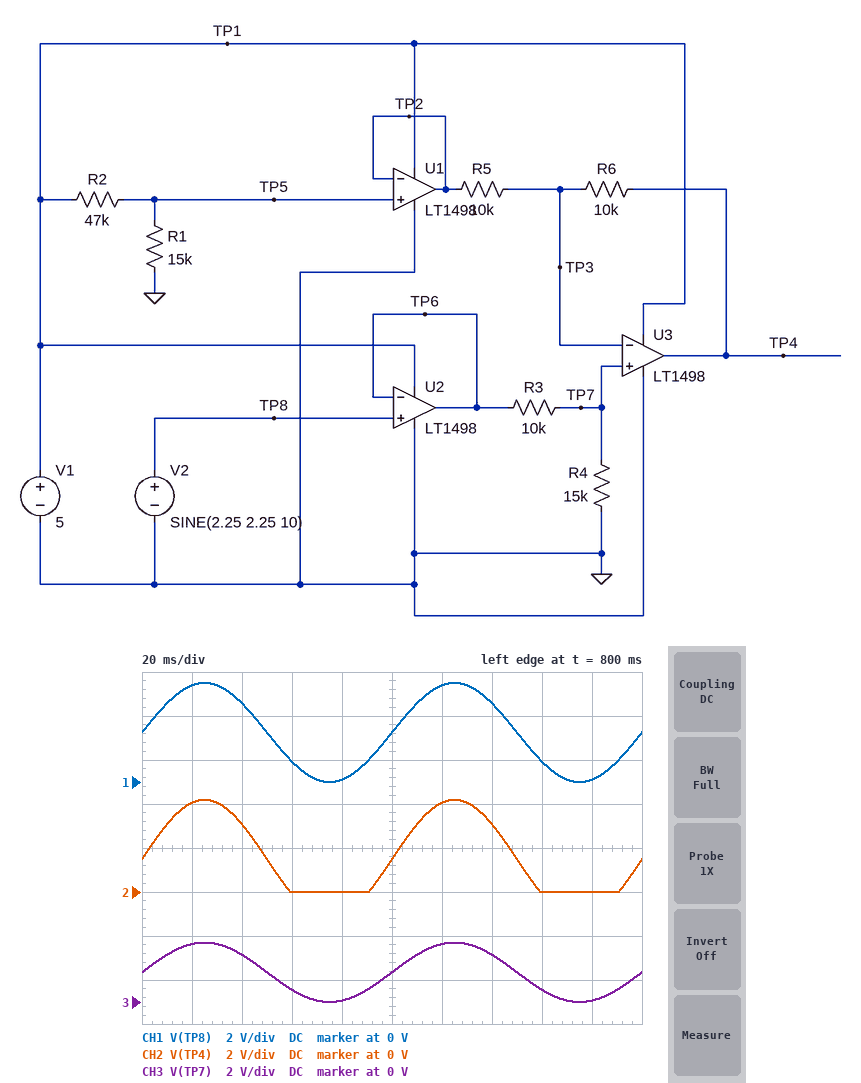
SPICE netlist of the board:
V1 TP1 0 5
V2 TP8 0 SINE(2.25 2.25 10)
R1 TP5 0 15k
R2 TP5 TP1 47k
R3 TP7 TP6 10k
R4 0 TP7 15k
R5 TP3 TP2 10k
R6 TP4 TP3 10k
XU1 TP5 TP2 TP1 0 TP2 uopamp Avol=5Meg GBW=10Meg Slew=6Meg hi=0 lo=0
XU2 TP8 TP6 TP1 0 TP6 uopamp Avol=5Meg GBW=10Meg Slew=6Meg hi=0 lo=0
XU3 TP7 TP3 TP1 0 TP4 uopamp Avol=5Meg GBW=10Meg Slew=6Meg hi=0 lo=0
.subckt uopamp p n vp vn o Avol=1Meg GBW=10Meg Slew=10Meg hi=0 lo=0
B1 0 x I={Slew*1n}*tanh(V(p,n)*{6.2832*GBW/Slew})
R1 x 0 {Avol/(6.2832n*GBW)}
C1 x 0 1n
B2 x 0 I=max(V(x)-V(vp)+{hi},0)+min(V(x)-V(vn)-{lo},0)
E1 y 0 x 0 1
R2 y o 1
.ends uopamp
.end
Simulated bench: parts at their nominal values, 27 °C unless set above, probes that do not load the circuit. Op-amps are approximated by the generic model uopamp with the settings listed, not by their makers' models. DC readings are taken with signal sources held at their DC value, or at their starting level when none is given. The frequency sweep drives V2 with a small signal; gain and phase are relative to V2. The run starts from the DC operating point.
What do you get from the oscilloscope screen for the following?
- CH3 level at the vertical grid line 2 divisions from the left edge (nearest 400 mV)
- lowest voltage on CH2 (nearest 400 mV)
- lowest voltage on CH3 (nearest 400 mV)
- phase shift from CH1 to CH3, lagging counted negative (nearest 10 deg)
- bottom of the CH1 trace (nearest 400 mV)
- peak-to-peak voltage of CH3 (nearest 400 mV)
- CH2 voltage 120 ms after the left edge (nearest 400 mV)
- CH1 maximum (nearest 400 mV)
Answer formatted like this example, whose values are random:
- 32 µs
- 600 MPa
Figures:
- 2.0 V
- 0 V
- 0 V
- 0 deg
- 0 V
- 2.8 V
- 4.0 V
- 4.4 V
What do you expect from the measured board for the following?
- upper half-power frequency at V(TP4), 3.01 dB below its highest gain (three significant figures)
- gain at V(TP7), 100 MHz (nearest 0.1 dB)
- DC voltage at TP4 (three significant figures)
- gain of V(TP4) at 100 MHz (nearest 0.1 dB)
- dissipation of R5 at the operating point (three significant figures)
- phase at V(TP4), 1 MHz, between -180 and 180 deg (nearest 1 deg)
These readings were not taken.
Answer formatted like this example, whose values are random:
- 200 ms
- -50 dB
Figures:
- 4.19 MHz
- -24.5 dB
- 1.49 V
- -44.5 dB
- 1.97 µW
- -17 deg
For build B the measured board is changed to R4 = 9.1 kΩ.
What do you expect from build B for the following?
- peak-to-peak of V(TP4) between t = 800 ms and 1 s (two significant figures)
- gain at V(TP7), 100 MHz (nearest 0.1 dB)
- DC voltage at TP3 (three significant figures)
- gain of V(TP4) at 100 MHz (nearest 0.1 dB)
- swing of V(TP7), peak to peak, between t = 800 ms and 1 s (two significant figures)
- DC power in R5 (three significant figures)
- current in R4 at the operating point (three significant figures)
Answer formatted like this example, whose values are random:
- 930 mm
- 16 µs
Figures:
- 3.1 V
- -26.5 dB
- 1.07 V
- -46.5 dB
- 2.1 V
- 1.90 µW
- 118 µA
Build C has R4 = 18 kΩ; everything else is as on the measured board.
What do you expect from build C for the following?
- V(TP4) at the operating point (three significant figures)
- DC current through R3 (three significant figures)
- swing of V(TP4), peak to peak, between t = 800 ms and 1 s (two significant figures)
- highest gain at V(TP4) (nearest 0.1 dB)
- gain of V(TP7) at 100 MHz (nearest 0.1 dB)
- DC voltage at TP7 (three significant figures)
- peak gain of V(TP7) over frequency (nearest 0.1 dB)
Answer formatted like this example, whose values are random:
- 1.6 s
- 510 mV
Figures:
- 1.68 V
- 80.4 µA
- 4.6 V
- 2.2 dB
- -23.9 dB
- 1.45 V
- -3.8 dB
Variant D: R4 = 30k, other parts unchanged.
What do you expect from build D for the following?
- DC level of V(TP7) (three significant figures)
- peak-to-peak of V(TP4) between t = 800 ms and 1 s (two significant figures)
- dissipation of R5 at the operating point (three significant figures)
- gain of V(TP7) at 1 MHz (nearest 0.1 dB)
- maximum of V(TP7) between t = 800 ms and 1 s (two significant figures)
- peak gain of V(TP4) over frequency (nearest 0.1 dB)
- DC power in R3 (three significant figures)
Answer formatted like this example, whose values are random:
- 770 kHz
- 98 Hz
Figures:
- 1.69 V
- 5.0 V
- 22.8 µW
- -2.5 dB
- 3.4 V
- 3.5 dB
- 31.6 µW
